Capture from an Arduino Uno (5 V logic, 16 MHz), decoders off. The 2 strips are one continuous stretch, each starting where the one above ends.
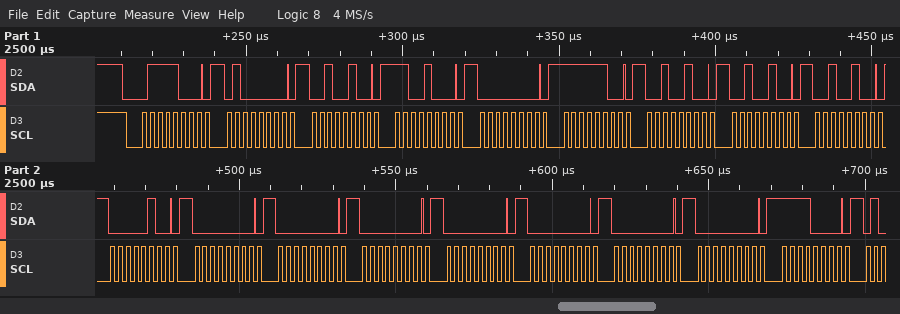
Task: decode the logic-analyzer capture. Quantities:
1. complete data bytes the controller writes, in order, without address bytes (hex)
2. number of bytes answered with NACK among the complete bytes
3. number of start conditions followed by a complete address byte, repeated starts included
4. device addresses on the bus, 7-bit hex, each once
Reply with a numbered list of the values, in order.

1. 40 24 C8 00 FC 24 24 24 04 00 00 00 00 00 00 00 F0
2. 0
3. 1
4. 0x3C
